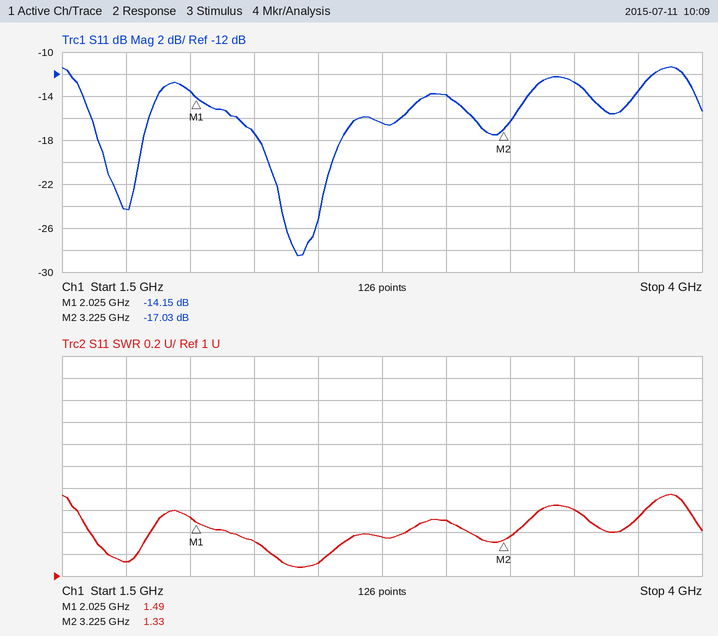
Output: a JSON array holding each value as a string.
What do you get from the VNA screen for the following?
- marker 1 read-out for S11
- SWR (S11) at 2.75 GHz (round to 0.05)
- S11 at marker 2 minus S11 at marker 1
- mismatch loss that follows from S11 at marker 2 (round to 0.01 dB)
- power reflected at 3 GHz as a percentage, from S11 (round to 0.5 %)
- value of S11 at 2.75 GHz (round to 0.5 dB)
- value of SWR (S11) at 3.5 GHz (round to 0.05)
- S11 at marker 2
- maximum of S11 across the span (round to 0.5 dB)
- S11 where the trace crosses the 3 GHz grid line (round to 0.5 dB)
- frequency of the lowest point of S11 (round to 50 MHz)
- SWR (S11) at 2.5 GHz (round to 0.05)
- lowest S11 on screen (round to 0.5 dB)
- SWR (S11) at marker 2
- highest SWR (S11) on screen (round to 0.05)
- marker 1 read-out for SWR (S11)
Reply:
["-14.15 dB", "1.35", "-2.88 dB", "0.09 dB", "4.0 %", "-16.5 dB", "1.60", "-17.03 dB", "-11.5 dB", "-14.0 dB", "2.40 GHz", "1.10", "-28.5 dB", "1.33", "1.75", "1.49"]
